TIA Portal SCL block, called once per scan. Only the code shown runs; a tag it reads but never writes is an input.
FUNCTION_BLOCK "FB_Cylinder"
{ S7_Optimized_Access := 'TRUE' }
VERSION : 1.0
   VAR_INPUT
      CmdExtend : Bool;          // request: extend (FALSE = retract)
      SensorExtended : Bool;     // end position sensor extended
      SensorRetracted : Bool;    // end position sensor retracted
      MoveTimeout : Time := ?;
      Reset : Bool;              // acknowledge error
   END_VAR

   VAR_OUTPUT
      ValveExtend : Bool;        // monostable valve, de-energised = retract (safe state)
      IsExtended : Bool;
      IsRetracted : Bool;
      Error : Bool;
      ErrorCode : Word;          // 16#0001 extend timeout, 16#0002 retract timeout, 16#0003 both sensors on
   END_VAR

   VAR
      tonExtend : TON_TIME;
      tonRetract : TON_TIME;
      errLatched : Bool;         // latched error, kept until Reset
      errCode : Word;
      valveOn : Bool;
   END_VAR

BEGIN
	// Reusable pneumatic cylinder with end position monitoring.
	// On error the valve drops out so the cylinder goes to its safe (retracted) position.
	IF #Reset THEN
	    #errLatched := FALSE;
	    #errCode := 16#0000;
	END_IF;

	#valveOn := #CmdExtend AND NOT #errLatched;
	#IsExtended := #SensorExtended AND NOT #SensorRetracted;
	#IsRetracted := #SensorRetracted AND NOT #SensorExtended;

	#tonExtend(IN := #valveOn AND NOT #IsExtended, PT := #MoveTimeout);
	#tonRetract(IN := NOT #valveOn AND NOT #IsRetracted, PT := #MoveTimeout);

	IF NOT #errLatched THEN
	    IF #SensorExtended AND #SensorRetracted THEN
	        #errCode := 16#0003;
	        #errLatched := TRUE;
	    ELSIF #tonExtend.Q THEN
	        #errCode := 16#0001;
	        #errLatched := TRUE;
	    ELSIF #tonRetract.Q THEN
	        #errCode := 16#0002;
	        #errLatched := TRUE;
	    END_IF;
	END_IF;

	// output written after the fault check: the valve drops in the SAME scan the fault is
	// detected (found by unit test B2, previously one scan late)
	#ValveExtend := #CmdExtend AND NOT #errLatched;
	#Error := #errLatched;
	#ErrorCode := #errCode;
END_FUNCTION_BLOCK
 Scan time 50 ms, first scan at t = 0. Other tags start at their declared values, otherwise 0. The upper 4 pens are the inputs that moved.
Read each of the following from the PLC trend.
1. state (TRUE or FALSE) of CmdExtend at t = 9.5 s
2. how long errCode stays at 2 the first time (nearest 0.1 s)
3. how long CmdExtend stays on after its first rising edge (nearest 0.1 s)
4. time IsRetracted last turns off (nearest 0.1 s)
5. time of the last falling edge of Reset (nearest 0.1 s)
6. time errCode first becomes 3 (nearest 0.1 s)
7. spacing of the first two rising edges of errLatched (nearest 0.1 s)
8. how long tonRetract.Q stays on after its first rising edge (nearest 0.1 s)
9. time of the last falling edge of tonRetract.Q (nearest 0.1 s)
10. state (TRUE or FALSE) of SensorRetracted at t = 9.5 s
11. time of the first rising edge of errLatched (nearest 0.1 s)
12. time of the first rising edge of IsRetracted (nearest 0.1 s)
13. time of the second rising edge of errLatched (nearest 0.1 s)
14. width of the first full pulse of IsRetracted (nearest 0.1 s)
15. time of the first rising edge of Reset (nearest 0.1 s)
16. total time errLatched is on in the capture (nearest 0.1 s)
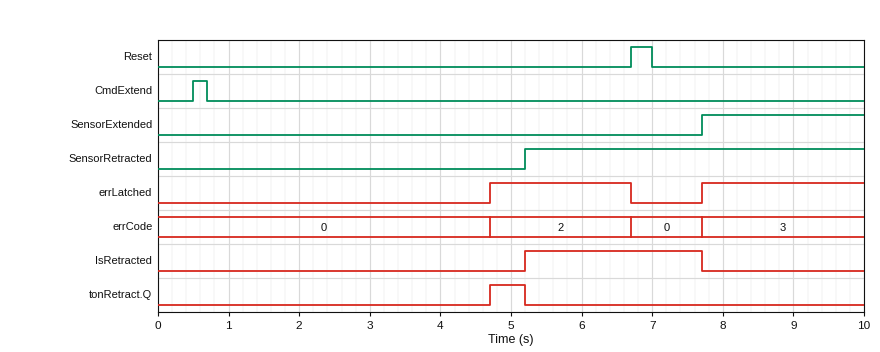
FALSE
2.0 s
0.2 s
7.7 s
7.0 s
7.7 s
3.0 s
0.5 s
5.2 s
TRUE
4.7 s
5.2 s
7.7 s
2.5 s
6.7 s
4.3 s
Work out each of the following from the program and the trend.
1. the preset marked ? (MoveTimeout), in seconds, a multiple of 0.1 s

4.0 s
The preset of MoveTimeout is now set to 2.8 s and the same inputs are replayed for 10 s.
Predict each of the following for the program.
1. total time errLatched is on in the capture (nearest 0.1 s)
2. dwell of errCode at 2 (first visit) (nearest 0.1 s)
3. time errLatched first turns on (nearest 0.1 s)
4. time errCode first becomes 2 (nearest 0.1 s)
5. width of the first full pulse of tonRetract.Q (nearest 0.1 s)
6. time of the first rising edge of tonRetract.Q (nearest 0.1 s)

5.5 s
3.2 s
3.5 s
3.5 s
1.7 s
3.5 s
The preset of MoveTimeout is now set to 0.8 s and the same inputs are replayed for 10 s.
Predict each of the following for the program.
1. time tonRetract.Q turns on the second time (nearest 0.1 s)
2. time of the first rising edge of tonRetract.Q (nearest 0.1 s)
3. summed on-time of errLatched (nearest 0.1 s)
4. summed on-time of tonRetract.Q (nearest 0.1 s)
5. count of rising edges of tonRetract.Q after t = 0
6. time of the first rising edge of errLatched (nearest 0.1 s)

8.5 s
1.5 s
7.5 s
5.2 s
2
1.5 s
